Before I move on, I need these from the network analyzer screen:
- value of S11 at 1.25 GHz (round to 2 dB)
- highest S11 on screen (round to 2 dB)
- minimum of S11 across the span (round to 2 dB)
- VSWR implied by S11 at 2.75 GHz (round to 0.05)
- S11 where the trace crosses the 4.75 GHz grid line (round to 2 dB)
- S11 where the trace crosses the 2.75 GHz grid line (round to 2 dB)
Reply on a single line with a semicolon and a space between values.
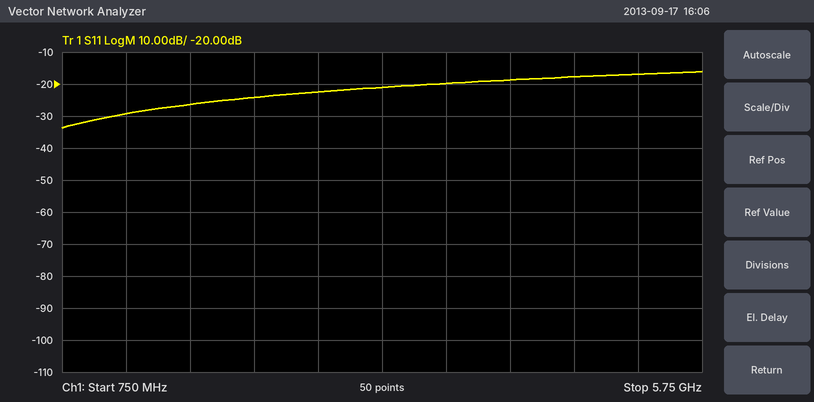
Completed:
-30 dB; -16 dB; -34 dB; 1.15; -18 dB; -22 dB
